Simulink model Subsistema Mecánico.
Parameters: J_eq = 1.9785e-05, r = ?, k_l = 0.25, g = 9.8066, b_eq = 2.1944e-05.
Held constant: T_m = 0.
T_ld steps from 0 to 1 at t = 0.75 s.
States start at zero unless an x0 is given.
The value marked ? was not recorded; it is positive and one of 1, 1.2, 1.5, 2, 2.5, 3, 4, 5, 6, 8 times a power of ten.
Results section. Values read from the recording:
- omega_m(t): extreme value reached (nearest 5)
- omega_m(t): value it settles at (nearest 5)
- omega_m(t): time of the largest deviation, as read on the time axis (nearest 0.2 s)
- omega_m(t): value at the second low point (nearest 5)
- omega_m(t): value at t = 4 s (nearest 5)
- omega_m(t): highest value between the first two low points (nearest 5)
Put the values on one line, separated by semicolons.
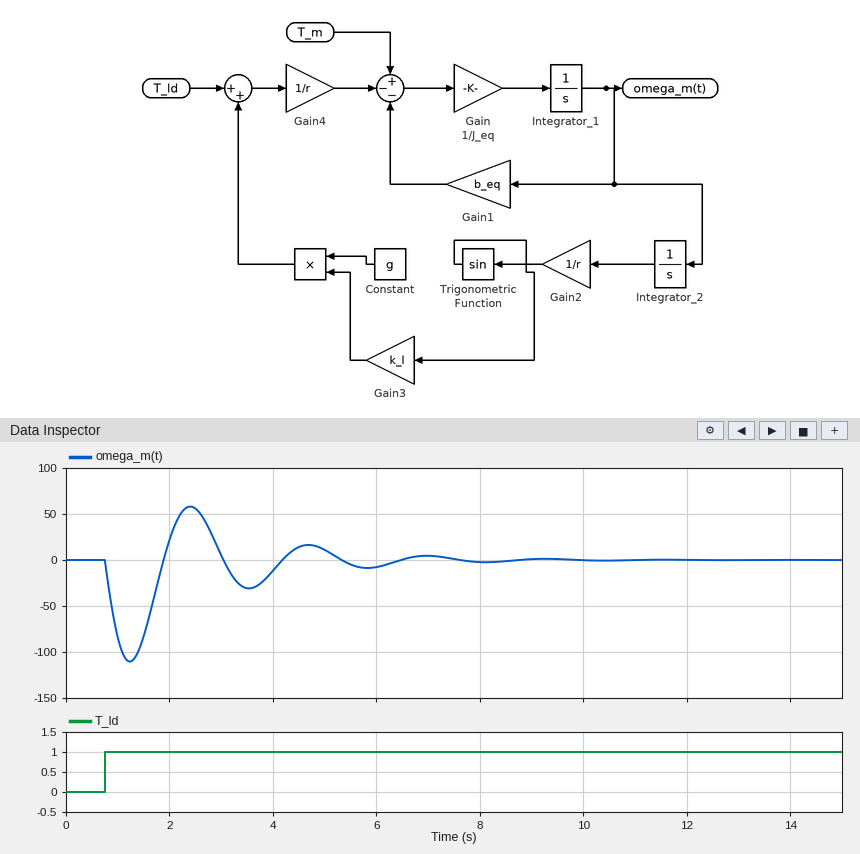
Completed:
-110; 0; 1.2 s; -30; -10; 60
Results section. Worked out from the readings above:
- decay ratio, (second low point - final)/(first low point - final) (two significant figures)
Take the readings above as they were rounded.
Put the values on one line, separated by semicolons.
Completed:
0.27
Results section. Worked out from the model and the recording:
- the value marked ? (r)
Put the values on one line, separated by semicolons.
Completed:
120
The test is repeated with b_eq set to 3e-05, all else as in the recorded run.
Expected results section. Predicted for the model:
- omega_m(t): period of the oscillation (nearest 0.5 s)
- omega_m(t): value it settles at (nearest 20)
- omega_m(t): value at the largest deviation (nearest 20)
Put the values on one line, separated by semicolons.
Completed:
2.5 s; 0; -100
